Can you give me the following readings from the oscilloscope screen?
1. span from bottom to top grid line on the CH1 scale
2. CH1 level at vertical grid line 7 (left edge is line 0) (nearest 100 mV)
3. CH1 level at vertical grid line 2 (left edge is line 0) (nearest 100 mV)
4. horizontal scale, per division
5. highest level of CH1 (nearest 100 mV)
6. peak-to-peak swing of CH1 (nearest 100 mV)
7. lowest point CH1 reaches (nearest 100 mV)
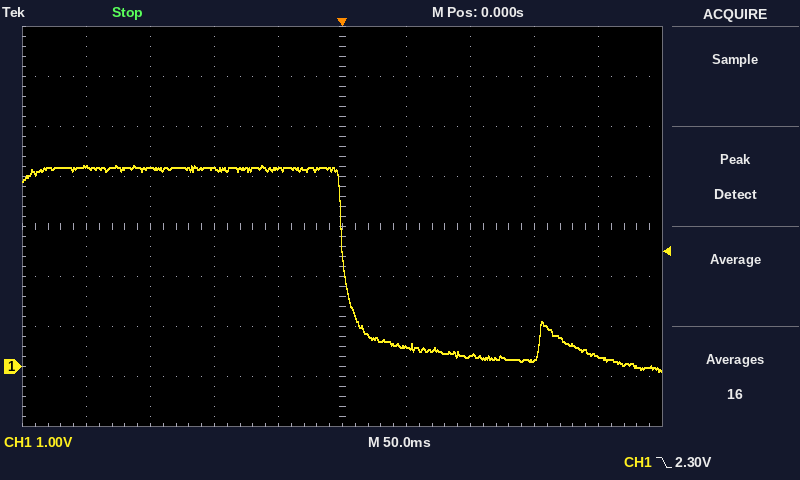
8 V
200 mV
4.0 V
50 ms
4.0 V
4.1 V
-100 mV
